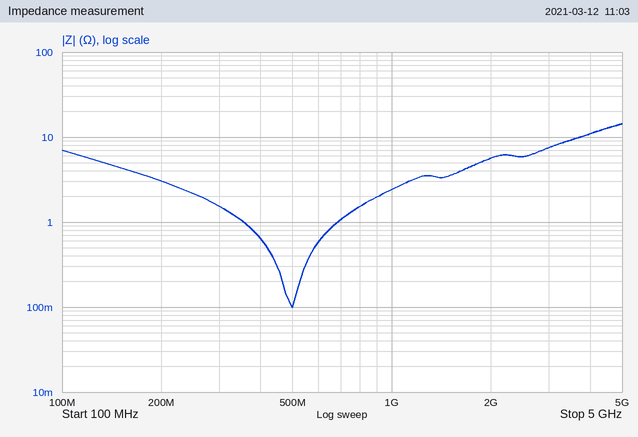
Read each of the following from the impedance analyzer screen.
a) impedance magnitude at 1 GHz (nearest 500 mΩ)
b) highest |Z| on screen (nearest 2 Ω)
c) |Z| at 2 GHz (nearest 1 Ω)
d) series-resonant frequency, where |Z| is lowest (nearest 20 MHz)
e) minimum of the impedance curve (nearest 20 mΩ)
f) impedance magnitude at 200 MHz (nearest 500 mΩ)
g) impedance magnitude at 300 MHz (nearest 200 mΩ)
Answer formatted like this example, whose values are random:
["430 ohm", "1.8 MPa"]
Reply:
["2.5 Ω", "14 Ω", "6 Ω", "500 MHz", "100 mΩ", "3.0 Ω", "1.6 Ω"]
